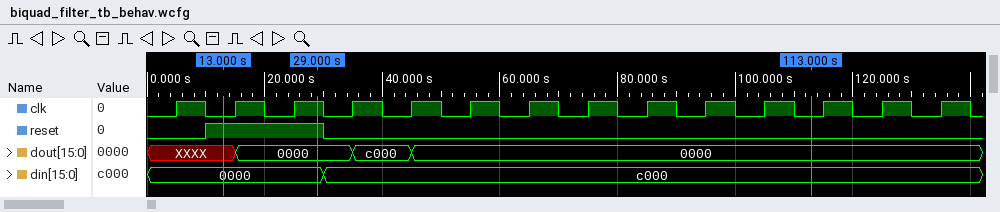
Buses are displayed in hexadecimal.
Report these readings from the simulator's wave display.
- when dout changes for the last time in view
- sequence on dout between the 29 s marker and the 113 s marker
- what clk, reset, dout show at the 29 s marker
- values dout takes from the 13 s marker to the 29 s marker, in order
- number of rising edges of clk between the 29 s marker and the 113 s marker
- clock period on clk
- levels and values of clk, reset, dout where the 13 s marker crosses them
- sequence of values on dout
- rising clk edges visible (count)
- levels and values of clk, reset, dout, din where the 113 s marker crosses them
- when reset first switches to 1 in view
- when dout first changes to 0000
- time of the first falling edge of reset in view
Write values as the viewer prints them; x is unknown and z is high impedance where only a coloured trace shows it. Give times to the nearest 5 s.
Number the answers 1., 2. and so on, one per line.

1. 45 s
2. 0000, c000, 0000
3. clk=1, reset=1, dout=0000
4. XXXX, 0000
5. 8
6. 10 s
7. clk=0, reset=1, dout=XXXX
8. XXXX, 0000, c000, 0000
9. 14
10. clk=0, reset=0, dout=0000, din=c000
11. 10 s
12. 15 s
13. 30 s
